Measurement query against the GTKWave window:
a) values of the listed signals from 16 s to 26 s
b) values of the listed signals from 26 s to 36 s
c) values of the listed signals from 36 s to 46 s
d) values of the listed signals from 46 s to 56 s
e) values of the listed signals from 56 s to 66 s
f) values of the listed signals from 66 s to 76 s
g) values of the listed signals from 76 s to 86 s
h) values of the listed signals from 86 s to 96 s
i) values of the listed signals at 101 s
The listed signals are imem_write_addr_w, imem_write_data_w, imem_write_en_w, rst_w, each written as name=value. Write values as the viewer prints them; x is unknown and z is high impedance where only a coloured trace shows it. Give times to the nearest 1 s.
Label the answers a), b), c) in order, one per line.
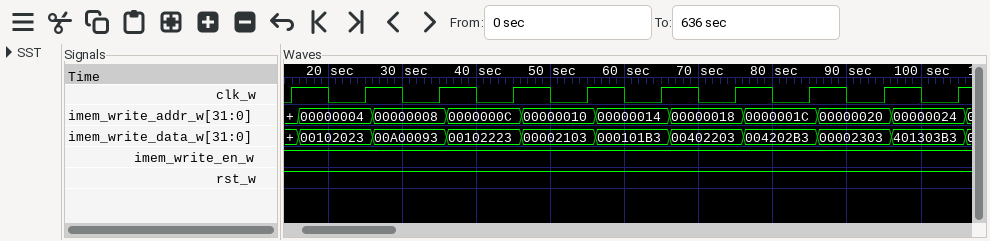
a) imem_write_addr_w=00000004, imem_write_data_w=00102023, imem_write_en_w=1, rst_w=1
b) imem_write_addr_w=00000008, imem_write_data_w=00A00093, imem_write_en_w=1, rst_w=1
c) imem_write_addr_w=0000000C, imem_write_data_w=00102223, imem_write_en_w=1, rst_w=1
d) imem_write_addr_w=00000010, imem_write_data_w=00002103, imem_write_en_w=1, rst_w=1
e) imem_write_addr_w=00000014, imem_write_data_w=000101B3, imem_write_en_w=1, rst_w=1
f) imem_write_addr_w=00000018, imem_write_data_w=00402203, imem_write_en_w=1, rst_w=1
g) imem_write_addr_w=0000001C, imem_write_data_w=004202B3, imem_write_en_w=1, rst_w=1
h) imem_write_addr_w=00000020, imem_write_data_w=00002303, imem_write_en_w=1, rst_w=1
i) imem_write_addr_w=00000024, imem_write_data_w=401303B3, imem_write_en_w=1, rst_w=1
